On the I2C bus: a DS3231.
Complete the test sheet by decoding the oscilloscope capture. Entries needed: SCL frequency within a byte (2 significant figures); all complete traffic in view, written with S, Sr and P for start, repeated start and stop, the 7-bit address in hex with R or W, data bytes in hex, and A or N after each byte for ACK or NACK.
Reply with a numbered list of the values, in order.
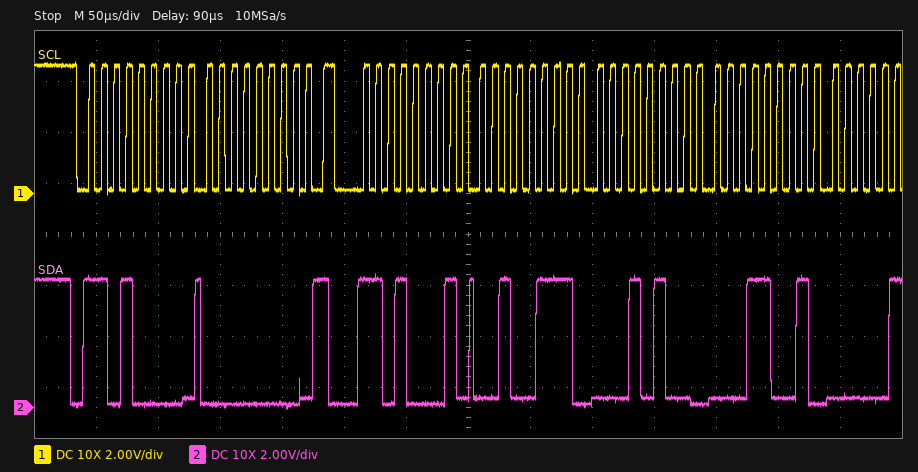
1. 100 kHz
2. S 68W A 00 A Sr 68R A 27 A 14 A 19 A
